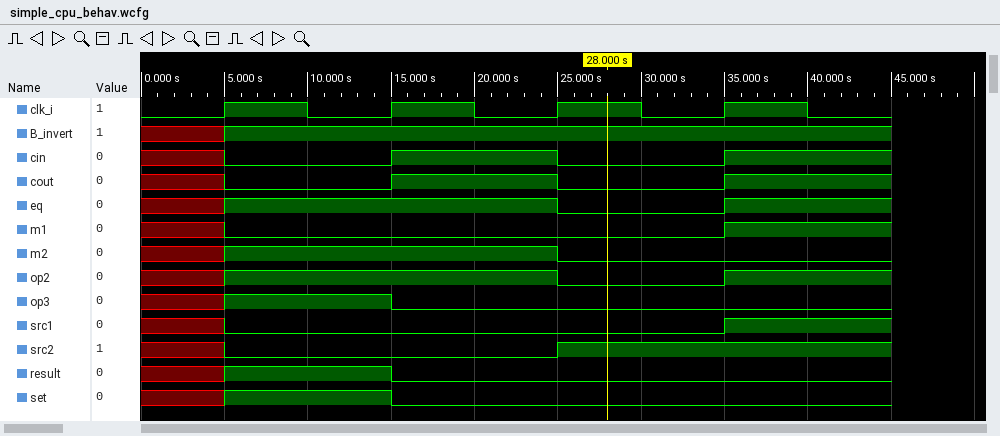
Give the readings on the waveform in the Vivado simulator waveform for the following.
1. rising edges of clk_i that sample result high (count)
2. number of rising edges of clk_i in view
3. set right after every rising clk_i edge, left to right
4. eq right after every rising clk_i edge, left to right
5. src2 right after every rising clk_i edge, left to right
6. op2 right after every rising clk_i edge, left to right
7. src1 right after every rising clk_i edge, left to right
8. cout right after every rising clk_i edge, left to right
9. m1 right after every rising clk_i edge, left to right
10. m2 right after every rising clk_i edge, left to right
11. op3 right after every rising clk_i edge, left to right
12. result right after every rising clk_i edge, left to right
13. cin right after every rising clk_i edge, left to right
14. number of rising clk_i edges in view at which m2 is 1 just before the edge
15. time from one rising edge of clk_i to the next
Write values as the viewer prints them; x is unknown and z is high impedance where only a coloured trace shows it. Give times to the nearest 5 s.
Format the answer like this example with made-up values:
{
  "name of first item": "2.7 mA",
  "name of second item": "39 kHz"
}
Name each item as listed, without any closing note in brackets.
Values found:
{
  "rising edges of clk_i that sample result high": "1",
  "number of rising edges of clk_i in view": "4",
  "set right after every rising clk_i edge, left to right": "1 0 0 0",
  "eq right after every rising clk_i edge, left to right": "1 1 0 1",
  "src2 right after every rising clk_i edge, left to right": "0 0 1 1",
  "op2 right after every rising clk_i edge, left to right": "1 1 0 1",
  "src1 right after every rising clk_i edge, left to right": "0 0 0 1",
  "cout right after every rising clk_i edge, left to right": "0 1 0 1",
  "m1 right after every rising clk_i edge, left to right": "0 0 0 1",
  "m2 right after every rising clk_i edge, left to right": "1 1 0 0",
  "op3 right after every rising clk_i edge, left to right": "1 0 0 0",
  "result right after every rising clk_i edge, left to right": "1 0 0 0",
  "cin right after every rising clk_i edge, left to right": "0 1 0 1",
  "number of rising clk_i edges in view at which m2 is 1 just before the edge": "2",
  "time from one rising edge of clk_i to the next": "10 s"
}
